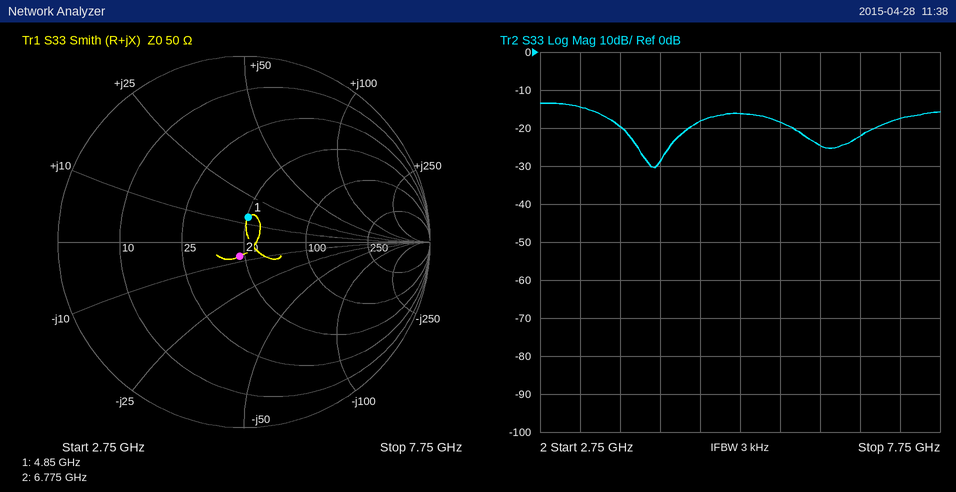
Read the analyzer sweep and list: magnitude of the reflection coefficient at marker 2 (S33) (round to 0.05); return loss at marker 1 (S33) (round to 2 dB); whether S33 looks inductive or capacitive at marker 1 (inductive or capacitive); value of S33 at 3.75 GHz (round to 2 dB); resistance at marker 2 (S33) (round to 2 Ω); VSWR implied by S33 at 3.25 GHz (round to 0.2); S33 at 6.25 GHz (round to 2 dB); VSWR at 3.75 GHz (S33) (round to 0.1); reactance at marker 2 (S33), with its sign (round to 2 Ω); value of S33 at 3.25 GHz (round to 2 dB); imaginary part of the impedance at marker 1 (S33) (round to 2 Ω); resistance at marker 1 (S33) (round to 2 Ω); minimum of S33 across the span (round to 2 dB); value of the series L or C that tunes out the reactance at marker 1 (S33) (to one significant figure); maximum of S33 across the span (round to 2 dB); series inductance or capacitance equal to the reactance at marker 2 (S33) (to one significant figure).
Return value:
0.10
18 dB
inductive
-20 dB
48 Ω
1.4
-24 dB
1.2
-8 Ω
-14 dB
+14 Ω
50 Ω
-30 dB
2 pF
-14 dB
3 pF
